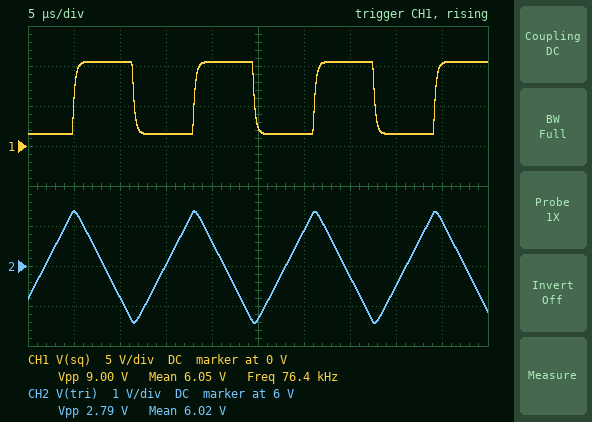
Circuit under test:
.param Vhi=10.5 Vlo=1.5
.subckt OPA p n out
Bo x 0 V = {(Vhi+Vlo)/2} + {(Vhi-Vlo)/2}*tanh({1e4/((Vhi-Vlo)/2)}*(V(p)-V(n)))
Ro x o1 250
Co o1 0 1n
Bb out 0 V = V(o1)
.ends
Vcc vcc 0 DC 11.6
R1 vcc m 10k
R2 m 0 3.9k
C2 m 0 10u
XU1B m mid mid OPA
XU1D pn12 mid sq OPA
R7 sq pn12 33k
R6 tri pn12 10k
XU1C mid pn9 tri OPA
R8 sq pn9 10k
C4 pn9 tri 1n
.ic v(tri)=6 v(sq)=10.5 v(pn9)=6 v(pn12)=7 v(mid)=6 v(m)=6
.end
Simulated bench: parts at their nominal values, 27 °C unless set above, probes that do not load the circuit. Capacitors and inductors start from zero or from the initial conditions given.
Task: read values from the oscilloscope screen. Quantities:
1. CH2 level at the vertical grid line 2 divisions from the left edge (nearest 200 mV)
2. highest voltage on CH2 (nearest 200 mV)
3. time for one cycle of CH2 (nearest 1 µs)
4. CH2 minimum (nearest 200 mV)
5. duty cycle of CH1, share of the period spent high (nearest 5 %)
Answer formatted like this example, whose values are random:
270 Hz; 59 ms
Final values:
5.2 V; 7.4 V; 13 µs; 4.6 V; 50 %
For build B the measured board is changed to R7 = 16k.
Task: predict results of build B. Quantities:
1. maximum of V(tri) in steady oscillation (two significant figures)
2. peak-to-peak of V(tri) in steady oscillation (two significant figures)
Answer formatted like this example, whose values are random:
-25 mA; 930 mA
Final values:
8.8 V; 5.7 V
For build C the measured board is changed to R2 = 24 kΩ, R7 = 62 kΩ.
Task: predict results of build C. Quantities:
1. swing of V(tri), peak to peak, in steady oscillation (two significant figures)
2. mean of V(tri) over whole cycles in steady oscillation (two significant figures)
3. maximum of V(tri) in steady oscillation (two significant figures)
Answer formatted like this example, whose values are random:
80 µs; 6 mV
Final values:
1.5 V; 6.0 V; 6.8 V
